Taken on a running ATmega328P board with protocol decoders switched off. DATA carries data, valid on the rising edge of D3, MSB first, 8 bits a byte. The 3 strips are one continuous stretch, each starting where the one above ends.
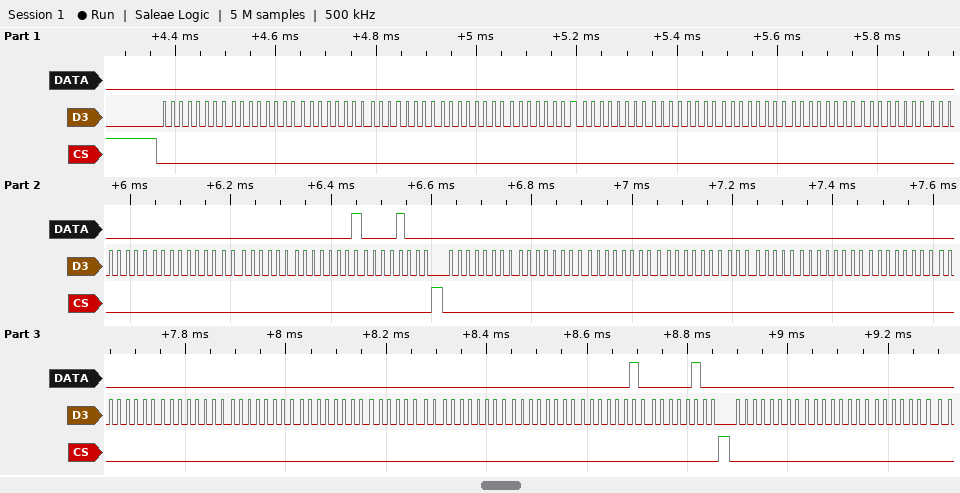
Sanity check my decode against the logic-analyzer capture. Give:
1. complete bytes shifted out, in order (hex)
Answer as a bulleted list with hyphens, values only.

- 00 00 00 00 00 00 00 00 00 00 00 00 00 00 01 08 00 00 00 00 00 00 00 00 00 00 00 00 00 00 02 04 00 00 00
